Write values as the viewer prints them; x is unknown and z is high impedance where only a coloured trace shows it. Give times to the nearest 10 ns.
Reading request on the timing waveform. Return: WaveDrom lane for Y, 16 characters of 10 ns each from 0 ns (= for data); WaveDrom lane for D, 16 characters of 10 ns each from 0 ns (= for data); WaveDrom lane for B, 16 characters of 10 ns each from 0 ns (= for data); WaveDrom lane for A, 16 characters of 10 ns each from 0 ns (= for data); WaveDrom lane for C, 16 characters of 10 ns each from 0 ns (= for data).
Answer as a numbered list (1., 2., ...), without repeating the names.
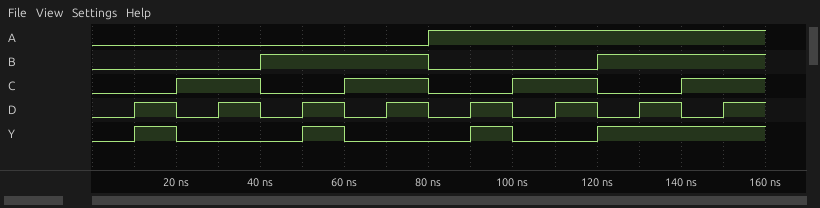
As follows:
1. {name: 'Y', wave: '010..10..10.1...'}
2. {name: 'D', wave: '0101010101010101'}
3. {name: 'B', wave: '0...1...0...1...'}
4. {name: 'A', wave: '0.......1.......'}
5. {name: 'C', wave: '0.1.0.1.0.1.0.1.'}
